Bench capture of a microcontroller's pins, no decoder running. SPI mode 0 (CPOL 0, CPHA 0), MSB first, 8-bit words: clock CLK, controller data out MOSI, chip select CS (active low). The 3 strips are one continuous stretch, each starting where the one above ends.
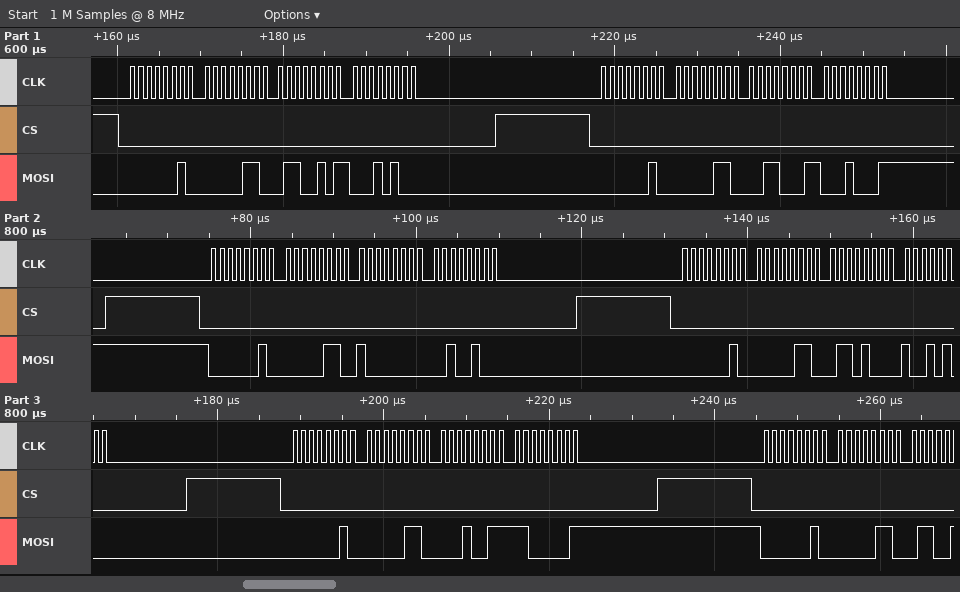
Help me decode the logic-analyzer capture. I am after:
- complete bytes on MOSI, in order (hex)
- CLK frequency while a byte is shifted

02 06 65 14 02 06 31 11 02 06 80 24 02 06 68 94 02 06 13 C1 02 06
1 MHz
